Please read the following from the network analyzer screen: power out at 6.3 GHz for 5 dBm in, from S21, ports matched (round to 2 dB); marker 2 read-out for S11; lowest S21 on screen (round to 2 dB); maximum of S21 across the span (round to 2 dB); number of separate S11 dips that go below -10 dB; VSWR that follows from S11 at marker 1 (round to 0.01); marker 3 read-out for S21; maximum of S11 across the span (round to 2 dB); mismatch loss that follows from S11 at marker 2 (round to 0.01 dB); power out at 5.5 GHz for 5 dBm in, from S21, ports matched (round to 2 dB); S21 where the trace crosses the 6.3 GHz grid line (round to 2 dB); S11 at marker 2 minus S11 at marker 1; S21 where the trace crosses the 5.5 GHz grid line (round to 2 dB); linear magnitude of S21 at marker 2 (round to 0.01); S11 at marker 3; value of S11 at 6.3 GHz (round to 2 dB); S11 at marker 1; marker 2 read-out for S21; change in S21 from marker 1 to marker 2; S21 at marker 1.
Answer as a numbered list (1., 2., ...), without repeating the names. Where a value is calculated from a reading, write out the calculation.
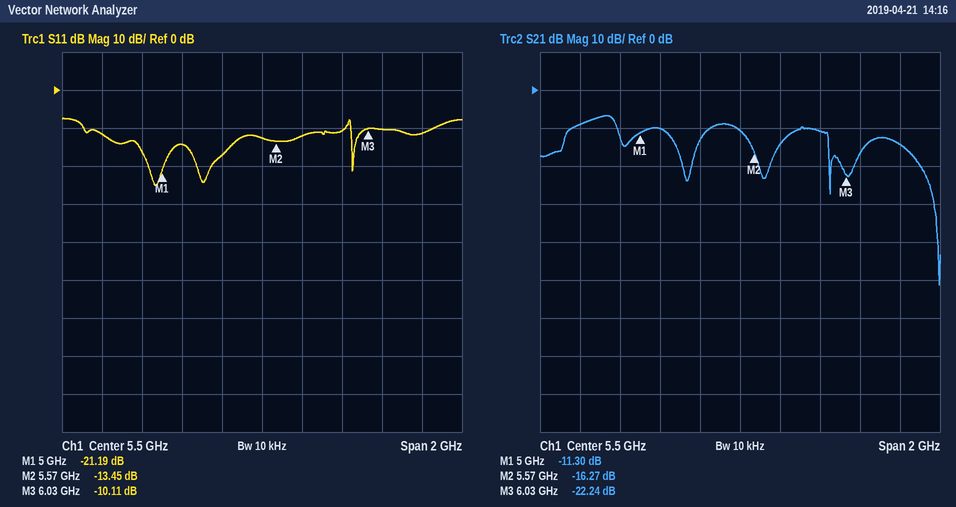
1. 5 dBm + (-14 dB) = -10 dBm
2. -13.45 dB
3. -52 dB
4. -6 dB
5. 3
6. (1 + 0.0872)/(1 − 0.0872) ≈ 1.19
7. -22.24 dB
8. -8 dB
9. −10 log10(1 − 10^(-13.45/10)) ≈ 0.20 dB
10. 5 dBm + (-10 dB) = -6 dBm
11. -14 dB
12. -13.45 − (-21.19) = 7.74 dB
13. -10 dB
14. 10^(-16.27/20) ≈ 0.15
15. -10.11 dB
16. -12 dB
17. -21.19 dB
18. -16.27 dB
19. -16.27 − (-11.3) = -4.97 dB
20. -11.30 dB
